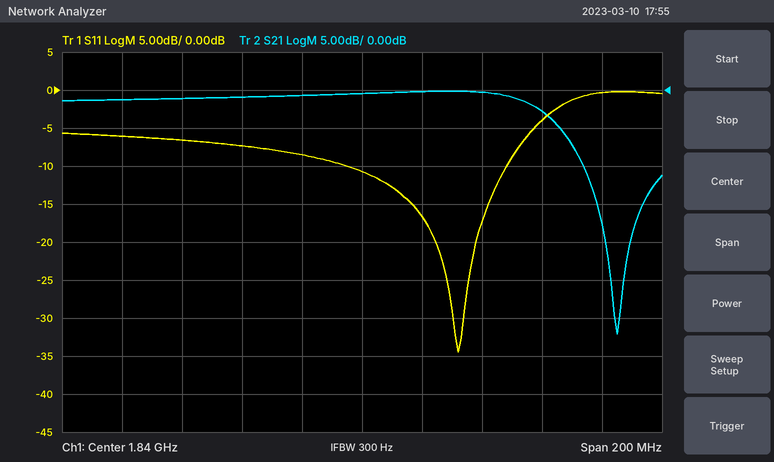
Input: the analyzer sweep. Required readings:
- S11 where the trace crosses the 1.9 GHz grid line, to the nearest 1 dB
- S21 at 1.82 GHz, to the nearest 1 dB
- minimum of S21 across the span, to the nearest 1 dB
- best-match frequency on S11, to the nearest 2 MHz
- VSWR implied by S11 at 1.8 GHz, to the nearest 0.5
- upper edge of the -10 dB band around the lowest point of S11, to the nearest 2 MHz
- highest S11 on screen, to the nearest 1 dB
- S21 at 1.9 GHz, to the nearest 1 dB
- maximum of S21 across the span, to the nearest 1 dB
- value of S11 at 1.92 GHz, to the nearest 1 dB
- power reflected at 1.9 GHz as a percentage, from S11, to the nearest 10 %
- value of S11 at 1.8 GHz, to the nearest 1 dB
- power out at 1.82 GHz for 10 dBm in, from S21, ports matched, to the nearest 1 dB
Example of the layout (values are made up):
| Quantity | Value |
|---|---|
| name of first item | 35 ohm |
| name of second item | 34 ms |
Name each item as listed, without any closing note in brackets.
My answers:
| Quantity | Value |
|---|---|
| S11 where the trace crosses the 1.9 GHz grid line, to the nearest 1 dB | -4 dB |
| S21 at 1.82 GHz, to the nearest 1 dB | -1 dB |
| minimum of S21 across the span, to the nearest 1 dB | -32 dB |
| best-match frequency on S11, to the nearest 2 MHz | 1.872 GHz |
| VSWR implied by S11 at 1.8 GHz, to the nearest 0.5 | 2.5 |
| upper edge of the -10 dB band around the lowest point of S11, to the nearest 2 MHz | 1.888 GHz |
| highest S11 on screen, to the nearest 1 dB | 0 dB |
| S21 at 1.9 GHz, to the nearest 1 dB | -3 dB |
| maximum of S21 across the span, to the nearest 1 dB | 0 dB |
| value of S11 at 1.92 GHz, to the nearest 1 dB | 0 dB |
| power reflected at 1.9 GHz as a percentage, from S11, to the nearest 10 % | 40 % |
| value of S11 at 1.8 GHz, to the nearest 1 dB | -7 dB |
| power out at 1.82 GHz for 10 dBm in, from S21, ports matched, to the nearest 1 dB | 9 dBm |
